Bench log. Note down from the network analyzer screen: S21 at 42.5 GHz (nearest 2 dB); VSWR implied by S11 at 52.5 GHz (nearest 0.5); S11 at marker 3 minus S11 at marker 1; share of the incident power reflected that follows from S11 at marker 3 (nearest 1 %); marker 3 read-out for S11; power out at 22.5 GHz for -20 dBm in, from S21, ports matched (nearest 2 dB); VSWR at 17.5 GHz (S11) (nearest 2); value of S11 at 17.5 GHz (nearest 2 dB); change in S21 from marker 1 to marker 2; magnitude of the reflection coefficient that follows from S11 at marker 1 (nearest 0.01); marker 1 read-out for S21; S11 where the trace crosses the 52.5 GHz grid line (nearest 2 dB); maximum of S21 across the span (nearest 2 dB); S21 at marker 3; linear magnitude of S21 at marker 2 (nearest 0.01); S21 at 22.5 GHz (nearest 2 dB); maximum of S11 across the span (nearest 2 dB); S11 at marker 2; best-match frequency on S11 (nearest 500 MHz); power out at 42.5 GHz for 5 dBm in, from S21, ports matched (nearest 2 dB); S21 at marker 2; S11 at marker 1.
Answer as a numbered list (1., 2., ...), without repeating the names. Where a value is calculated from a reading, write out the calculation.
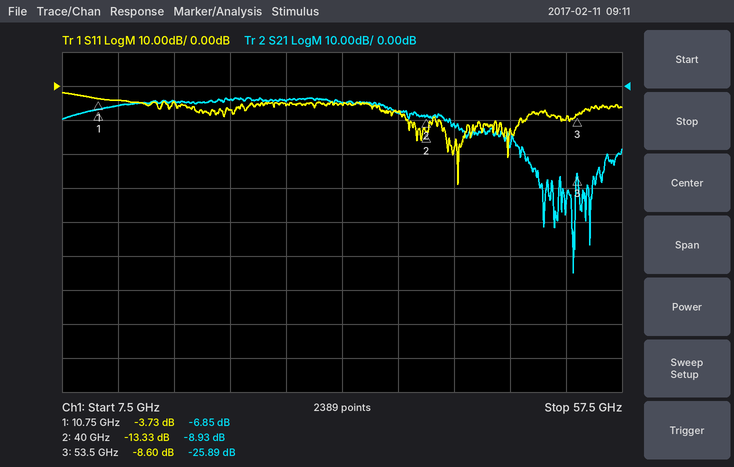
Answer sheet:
1. -12 dB
2. |Γ| = 10^(-10/20) = 0.3162; VSWR = (1 + 0.3162)/(1 − 0.3162) ≈ 1.92, so 2.0 to the nearest 0.5
3. -8.6 − (-3.73) = -4.87 dB
4. 10^(-8.6/10) ≈ 14 %
5. -8.60 dB
6. -20 dBm + (-4 dB) = -24 dBm
7. |Γ| = 10^(-4/20) = 0.6310; VSWR = (1 + 0.6310)/(1 − 0.6310) ≈ 4
8. -4 dB
9. -8.93 − (-6.85) = -2.08 dB
10. 10^(-3.73/20) ≈ 0.65
11. -6.85 dB
12. -10 dB
13. -4 dB
14. -25.89 dB
15. 10^(-8.93/20) ≈ 0.36
16. -4 dB
17. -2 dB
18. -13.33 dB
19. 43.0 GHz
20. 5 dBm + (-12 dB) = -6 dBm
21. -8.93 dB
22. -3.73 dB
